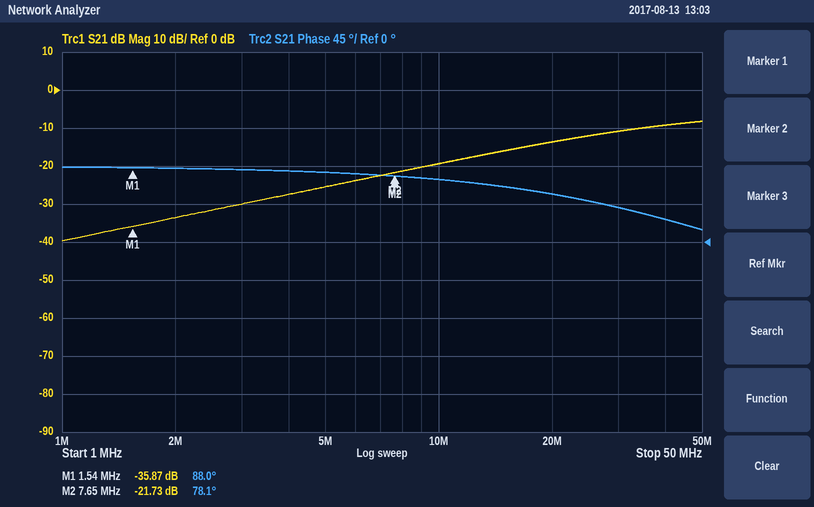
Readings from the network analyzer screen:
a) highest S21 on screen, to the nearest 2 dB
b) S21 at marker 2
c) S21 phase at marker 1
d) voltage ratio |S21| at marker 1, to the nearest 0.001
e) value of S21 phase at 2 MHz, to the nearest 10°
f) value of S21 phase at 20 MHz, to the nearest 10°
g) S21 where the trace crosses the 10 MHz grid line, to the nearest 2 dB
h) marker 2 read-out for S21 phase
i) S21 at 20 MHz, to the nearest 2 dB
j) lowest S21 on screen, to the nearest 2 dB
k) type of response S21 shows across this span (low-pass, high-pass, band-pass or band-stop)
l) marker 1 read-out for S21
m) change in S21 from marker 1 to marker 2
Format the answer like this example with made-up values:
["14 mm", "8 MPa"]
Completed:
["-8 dB", "-21.73 dB", "88.0°", "0.016", "90°", "60°", "-20 dB", "78.1°", "-14 dB", "-40 dB", "high-pass", "-35.87 dB", "14.14 dB"]
